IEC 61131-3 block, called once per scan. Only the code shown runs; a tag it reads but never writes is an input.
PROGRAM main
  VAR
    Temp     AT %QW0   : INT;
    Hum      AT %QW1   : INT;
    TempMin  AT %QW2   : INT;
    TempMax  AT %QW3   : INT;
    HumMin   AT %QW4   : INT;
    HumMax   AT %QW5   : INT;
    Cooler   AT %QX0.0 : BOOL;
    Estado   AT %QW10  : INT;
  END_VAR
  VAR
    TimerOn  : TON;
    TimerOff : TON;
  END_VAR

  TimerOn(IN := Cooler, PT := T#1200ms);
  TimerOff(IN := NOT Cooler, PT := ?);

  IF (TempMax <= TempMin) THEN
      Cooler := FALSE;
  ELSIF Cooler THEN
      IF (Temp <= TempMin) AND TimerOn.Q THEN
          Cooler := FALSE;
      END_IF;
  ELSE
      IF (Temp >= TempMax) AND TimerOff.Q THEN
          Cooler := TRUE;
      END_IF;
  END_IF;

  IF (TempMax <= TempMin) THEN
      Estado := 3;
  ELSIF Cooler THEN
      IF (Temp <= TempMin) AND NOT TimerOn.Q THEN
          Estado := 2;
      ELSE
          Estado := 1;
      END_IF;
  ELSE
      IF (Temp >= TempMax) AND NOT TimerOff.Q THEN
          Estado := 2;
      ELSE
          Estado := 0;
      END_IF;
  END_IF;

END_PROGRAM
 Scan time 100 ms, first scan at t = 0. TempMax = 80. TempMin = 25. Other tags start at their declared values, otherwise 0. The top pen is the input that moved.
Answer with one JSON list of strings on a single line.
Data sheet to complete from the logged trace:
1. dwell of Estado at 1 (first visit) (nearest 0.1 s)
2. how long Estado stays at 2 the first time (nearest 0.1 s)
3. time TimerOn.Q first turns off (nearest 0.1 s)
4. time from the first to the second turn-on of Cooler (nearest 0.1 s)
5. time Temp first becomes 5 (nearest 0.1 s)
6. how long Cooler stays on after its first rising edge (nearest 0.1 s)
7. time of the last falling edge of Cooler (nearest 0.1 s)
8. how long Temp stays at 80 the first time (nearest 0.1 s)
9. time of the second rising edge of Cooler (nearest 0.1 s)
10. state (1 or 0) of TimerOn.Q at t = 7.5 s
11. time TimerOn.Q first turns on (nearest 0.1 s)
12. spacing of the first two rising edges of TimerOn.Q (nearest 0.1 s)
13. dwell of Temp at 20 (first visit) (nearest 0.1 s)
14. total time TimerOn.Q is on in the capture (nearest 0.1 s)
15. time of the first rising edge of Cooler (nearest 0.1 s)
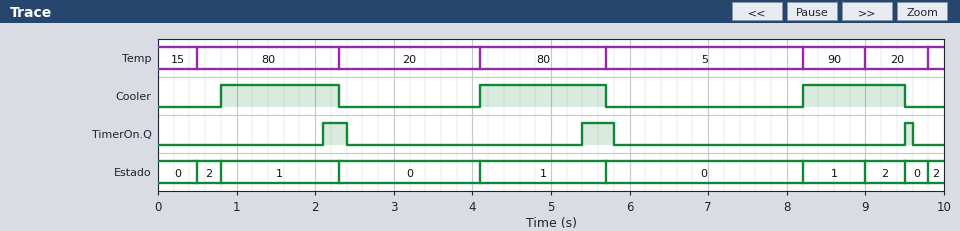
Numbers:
["1.5 s", "0.3 s", "2.4 s", "3.3 s", "5.7 s", "1.5 s", "9.5 s", "1.8 s", "4.1 s", "0", "2.1 s", "3.3 s", "1.8 s", "0.8 s", "0.8 s"]
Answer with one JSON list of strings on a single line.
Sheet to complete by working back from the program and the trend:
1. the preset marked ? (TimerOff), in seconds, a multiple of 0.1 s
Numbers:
["0.8 s"]
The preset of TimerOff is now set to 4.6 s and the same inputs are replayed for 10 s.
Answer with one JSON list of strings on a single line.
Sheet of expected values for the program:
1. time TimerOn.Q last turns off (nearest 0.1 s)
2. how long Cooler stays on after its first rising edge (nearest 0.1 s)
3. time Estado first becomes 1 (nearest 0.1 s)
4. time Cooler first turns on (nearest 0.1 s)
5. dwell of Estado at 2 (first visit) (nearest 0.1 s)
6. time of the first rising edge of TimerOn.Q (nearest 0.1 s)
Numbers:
["6.0 s", "1.3 s", "4.6 s", "4.6 s", "1.8 s", "5.9 s"]
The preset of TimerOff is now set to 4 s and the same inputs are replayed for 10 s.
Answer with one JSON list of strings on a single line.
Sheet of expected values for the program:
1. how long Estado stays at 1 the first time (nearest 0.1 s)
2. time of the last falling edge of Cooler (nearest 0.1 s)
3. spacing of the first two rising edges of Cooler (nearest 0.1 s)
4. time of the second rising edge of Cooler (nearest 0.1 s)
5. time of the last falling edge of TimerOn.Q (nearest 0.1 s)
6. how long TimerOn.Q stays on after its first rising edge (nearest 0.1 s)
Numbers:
["1.6 s", "5.7 s", "5.7 s", "9.8 s", "5.8 s", "0.4 s"]
